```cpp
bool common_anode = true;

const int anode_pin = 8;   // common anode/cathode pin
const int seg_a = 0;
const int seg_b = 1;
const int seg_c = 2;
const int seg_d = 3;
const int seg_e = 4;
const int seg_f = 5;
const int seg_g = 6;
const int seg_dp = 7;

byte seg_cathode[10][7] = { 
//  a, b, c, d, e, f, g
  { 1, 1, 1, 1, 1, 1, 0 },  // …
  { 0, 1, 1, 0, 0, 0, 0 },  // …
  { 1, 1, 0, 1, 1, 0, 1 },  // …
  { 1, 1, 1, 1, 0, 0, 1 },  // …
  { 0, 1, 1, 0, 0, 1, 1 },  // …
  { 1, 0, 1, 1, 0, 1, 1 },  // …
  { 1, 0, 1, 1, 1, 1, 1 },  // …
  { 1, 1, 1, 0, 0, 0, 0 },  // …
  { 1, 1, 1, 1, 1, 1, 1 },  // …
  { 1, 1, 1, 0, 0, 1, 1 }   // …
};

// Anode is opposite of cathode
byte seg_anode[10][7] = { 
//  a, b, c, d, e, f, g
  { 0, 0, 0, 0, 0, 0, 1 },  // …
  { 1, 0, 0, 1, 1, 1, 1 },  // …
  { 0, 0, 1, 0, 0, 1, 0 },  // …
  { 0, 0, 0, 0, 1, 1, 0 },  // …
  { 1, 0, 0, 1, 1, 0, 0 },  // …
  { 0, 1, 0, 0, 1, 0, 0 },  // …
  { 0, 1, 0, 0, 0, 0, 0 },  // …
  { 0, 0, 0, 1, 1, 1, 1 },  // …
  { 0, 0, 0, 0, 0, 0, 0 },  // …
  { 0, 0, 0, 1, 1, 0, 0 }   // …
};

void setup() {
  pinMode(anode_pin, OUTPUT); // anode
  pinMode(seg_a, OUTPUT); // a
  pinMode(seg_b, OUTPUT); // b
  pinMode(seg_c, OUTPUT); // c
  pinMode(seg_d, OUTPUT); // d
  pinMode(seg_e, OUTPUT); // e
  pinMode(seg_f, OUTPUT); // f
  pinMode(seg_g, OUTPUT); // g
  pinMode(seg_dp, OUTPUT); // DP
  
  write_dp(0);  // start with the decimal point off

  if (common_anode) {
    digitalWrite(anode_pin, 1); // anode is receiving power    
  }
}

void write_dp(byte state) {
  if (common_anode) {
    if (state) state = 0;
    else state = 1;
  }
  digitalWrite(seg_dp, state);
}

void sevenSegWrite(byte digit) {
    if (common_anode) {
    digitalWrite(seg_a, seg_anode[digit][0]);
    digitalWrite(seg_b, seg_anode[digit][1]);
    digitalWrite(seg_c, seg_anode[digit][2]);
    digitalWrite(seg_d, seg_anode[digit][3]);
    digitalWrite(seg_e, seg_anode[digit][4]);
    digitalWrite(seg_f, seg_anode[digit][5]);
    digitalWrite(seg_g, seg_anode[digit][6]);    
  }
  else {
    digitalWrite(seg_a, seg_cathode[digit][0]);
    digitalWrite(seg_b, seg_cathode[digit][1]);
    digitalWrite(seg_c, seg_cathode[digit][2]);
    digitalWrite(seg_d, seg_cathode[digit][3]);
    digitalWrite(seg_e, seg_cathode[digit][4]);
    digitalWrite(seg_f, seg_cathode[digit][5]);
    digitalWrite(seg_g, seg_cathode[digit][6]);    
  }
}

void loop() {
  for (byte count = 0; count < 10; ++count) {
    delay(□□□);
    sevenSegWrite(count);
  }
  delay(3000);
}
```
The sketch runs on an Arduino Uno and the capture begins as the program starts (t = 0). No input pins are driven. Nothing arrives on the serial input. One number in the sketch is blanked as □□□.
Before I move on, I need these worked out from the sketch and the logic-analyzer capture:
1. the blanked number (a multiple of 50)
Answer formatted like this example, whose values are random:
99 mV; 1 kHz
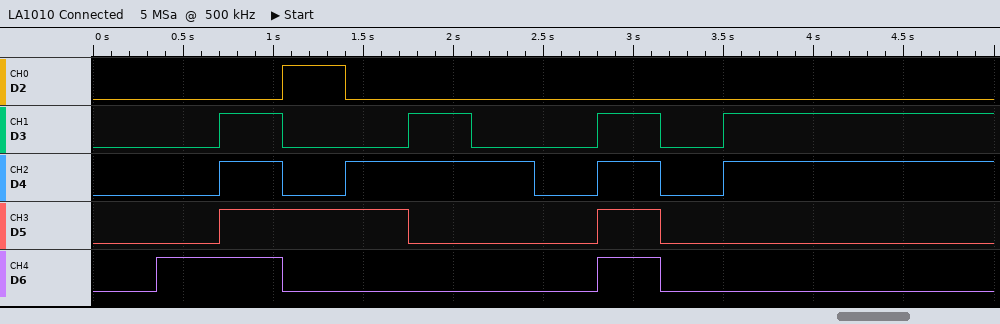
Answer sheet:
350
